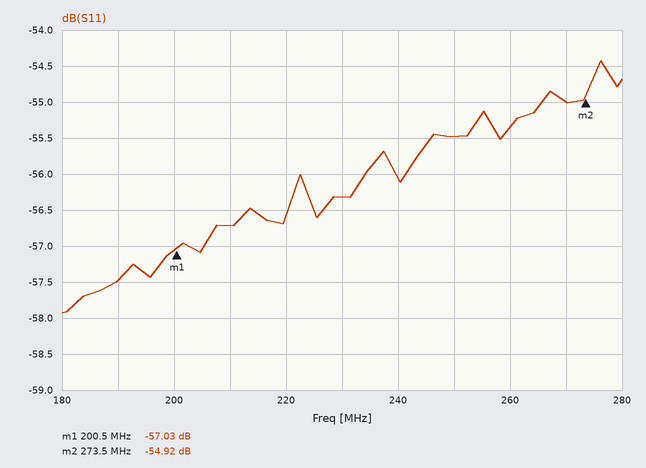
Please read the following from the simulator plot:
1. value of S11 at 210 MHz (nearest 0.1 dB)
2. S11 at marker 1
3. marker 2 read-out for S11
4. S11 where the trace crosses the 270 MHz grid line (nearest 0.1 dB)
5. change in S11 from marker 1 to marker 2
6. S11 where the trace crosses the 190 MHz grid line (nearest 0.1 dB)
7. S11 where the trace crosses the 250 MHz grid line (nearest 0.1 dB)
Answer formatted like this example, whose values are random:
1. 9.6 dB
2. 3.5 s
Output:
1. -56.7 dB
2. -57.03 dB
3. -54.92 dB
4. -55.0 dB
5. 2.11 dB
6. -57.5 dB
7. -55.5 dB
